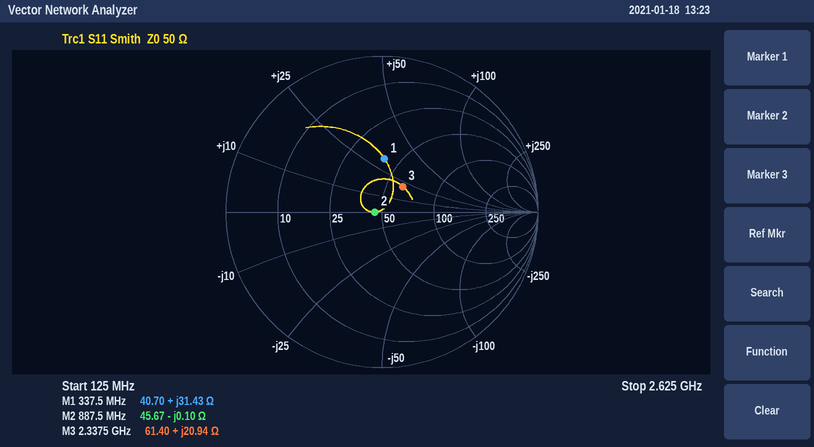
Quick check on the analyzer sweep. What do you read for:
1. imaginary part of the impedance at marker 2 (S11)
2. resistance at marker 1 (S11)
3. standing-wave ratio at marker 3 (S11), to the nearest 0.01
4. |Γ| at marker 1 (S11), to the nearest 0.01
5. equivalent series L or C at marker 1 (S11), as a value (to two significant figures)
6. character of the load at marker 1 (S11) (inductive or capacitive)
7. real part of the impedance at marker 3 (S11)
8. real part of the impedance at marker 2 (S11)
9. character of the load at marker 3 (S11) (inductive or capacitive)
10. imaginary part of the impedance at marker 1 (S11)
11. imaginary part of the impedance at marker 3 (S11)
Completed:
-0.10 Ω
40.70 Ω
1.53
0.34
15 nH
inductive
61.40 Ω
45.67 Ω
inductive
+31.43 Ω
+20.94 Ω
